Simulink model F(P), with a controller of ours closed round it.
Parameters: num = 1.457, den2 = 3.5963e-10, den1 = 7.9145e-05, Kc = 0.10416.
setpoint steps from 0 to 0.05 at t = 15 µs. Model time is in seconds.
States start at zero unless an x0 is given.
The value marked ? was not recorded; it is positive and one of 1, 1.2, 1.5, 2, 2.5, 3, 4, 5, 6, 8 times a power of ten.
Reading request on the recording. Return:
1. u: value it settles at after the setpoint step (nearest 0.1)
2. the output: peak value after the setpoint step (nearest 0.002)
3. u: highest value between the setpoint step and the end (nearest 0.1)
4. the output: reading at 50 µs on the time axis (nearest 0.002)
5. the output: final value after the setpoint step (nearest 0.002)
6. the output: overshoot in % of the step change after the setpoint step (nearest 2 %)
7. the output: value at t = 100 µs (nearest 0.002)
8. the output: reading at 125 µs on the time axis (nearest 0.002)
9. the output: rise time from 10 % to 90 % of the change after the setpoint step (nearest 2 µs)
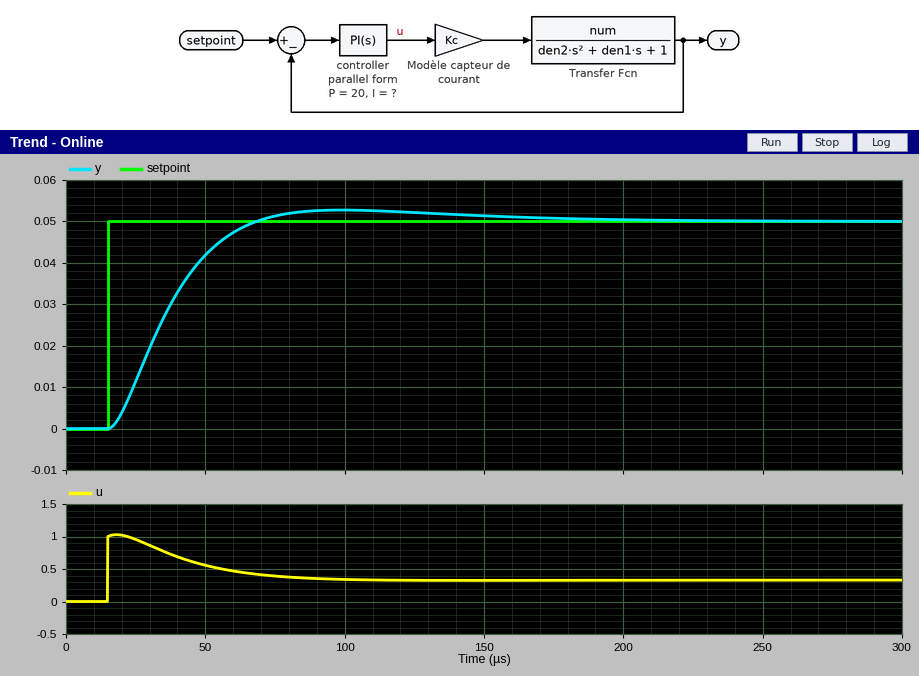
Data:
0.3
0.052
1.0
0.042
0.050
6 %
0.052
0.052
34 µs
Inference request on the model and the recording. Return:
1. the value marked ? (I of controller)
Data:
400000
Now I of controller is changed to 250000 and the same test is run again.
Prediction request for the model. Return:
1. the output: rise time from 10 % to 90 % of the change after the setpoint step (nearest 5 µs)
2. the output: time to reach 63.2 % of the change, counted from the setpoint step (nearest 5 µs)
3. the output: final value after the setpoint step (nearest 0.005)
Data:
45 µs
25 µs
0.050
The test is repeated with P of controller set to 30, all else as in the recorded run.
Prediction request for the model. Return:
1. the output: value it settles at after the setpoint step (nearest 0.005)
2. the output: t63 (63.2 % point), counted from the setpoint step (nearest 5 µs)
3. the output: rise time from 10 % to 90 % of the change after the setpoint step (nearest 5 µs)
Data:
0.050
20 µs
25 µs
